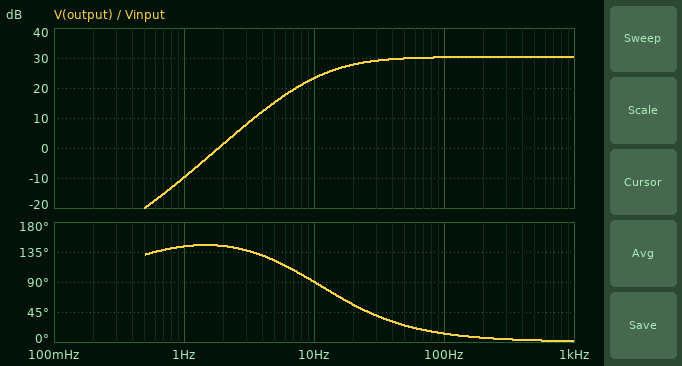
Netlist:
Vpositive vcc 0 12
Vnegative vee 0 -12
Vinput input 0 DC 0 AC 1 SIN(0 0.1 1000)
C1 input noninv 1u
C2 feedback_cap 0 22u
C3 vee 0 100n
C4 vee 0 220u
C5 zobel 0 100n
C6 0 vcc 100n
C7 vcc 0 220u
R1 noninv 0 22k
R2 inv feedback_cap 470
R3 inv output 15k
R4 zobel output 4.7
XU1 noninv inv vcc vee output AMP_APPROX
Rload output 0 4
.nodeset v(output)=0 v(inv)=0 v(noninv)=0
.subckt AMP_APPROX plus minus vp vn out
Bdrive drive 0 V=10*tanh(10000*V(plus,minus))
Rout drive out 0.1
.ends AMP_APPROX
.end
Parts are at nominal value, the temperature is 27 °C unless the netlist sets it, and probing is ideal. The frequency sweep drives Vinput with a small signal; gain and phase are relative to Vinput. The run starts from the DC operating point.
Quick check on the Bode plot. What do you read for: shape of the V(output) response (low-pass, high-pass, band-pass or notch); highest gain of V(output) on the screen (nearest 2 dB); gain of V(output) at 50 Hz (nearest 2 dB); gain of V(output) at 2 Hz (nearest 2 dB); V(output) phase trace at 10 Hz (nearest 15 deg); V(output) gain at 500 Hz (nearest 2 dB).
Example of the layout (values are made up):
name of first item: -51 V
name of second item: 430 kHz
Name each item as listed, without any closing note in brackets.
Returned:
shape of the V(output) response: high-pass
highest gain of V(output) on the screen: 30 dB
gain of V(output) at 50 Hz: 30 dB
gain of V(output) at 2 Hz: 2 dB
V(output) phase trace at 10 Hz: 90 deg
V(output) gain at 500 Hz: 30 dB
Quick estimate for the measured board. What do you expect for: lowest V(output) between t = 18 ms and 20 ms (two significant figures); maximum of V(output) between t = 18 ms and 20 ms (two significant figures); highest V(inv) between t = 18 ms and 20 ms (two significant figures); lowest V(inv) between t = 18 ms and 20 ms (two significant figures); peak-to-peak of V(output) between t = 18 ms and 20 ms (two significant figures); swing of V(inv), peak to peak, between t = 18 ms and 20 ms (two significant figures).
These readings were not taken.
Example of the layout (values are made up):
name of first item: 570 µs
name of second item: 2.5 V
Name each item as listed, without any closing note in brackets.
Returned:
lowest V(output) between t = 18 ms and 20 ms: -3.3 V
maximum of V(output) between t = 18 ms and 20 ms: 3.3 V
highest V(inv) between t = 18 ms and 20 ms: 100 mV
lowest V(inv) between t = 18 ms and 20 ms: -100 mV
peak-to-peak of V(output) between t = 18 ms and 20 ms: 6.6 V
swing of V(inv), peak to peak, between t = 18 ms and 20 ms: 200 mV
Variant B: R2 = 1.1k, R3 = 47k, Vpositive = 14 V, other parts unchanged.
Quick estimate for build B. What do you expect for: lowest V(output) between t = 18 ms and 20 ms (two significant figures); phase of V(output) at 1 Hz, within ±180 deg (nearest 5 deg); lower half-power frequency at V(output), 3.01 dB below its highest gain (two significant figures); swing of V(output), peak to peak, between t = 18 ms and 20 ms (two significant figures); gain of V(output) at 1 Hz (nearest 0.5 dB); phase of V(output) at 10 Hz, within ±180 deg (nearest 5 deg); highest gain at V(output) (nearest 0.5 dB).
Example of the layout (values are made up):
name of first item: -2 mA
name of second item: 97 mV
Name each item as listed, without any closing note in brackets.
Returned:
lowest V(output) between t = 18 ms and 20 ms: -4.4 V
phase of V(output) at 1 Hz, within ±180 deg: 155 deg
lower half-power frequency at V(output), 3.01 dB below its highest gain: 11 Hz
swing of V(output), peak to peak, between t = 18 ms and 20 ms: 8.7 V
gain of V(output) at 1 Hz: -1.0 dB
phase of V(output) at 10 Hz, within ±180 deg: 70 deg
highest gain at V(output): 33.0 dB
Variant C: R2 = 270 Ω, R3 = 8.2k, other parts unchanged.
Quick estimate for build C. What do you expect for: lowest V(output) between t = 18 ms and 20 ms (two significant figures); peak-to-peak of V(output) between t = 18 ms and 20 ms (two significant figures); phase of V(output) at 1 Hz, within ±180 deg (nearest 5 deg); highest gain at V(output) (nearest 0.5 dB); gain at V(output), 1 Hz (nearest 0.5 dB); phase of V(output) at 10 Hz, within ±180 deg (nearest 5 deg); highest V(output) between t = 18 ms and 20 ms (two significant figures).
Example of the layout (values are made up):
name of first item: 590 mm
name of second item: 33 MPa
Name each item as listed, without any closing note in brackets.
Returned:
lowest V(output) between t = 18 ms and 20 ms: -3.1 V
peak-to-peak of V(output) between t = 18 ms and 20 ms: 6.3 V
phase of V(output) at 1 Hz, within ±180 deg: 130 deg
highest gain at V(output): 30.0 dB
gain at V(output), 1 Hz: -13.5 dB
phase of V(output) at 10 Hz, within ±180 deg: 100 deg
highest V(output) between t = 18 ms and 20 ms: 3.1 V
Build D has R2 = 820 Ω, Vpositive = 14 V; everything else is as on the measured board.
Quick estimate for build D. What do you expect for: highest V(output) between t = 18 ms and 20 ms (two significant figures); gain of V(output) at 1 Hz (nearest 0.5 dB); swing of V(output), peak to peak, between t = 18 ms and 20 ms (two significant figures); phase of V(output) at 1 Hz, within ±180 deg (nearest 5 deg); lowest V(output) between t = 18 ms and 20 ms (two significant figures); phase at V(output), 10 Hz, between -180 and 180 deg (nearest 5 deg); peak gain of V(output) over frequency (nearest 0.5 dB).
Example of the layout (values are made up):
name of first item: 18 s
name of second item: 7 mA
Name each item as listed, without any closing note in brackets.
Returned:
highest V(output) between t = 18 ms and 20 ms: 1.9 V
gain of V(output) at 1 Hz: -9.5 dB
swing of V(output), peak to peak, between t = 18 ms and 20 ms: 3.9 V
phase of V(output) at 1 Hz, within ±180 deg: 140 deg
lowest V(output) between t = 18 ms and 20 ms: -1.9 V
phase at V(output), 10 Hz, between -180 and 180 deg: 75 deg
peak gain of V(output) over frequency: 25.5 dB
